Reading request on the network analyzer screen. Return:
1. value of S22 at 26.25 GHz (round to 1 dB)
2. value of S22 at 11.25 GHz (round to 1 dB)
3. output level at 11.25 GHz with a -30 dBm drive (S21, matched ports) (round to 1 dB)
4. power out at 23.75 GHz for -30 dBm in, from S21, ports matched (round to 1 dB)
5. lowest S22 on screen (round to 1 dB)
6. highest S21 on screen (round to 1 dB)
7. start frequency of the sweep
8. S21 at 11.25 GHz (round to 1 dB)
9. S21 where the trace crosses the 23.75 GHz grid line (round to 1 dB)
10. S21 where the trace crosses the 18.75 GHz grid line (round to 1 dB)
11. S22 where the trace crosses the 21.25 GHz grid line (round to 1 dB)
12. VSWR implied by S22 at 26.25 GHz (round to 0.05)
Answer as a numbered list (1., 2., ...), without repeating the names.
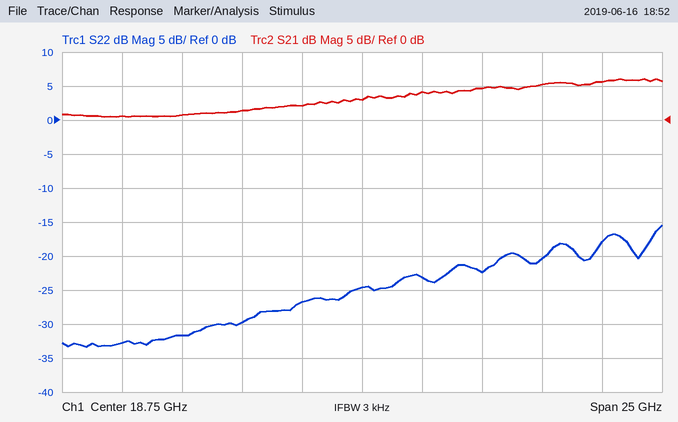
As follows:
1. -20 dB
2. -32 dB
3. -29 dBm
4. -25 dBm
5. -33 dB
6. 6 dB
7. 6.25 GHz
8. 1 dB
9. 5 dB
10. 3 dB
11. -23 dB
12. 1.20
